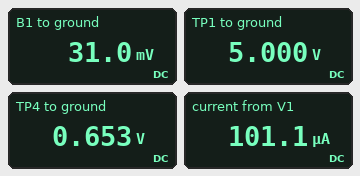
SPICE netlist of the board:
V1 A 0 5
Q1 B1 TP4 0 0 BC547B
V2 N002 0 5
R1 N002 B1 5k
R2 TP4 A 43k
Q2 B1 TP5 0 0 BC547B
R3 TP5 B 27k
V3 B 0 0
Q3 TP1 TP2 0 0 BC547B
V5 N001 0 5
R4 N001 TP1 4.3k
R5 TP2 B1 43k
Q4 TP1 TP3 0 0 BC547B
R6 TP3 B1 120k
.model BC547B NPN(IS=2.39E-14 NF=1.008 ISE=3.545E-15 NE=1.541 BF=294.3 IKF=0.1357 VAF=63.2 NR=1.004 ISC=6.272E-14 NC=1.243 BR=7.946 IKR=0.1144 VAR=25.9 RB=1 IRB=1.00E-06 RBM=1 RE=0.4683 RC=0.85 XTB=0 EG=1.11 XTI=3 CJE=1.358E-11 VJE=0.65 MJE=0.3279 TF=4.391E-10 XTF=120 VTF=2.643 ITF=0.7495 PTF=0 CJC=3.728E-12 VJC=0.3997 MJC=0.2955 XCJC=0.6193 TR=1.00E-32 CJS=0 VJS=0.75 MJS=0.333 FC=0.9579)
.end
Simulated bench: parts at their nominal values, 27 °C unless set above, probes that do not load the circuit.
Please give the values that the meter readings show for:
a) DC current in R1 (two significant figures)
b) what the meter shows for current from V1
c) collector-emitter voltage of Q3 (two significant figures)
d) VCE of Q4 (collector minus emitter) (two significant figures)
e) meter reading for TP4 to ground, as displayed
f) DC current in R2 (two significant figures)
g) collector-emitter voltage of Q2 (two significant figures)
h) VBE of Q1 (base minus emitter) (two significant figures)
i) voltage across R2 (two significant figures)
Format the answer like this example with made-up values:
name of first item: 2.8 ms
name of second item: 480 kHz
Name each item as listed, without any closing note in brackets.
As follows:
DC current in R1: 990 µA
what the meter shows for current from V1: 101.1 µA
collector-emitter voltage of Q3: 5.0 V
VCE of Q4 (collector minus emitter): 5.0 V
meter reading for TP4 to ground, as displayed: 0.653 V
DC current in R2: 100 µA
collector-emitter voltage of Q2: 31 mV
VBE of Q1 (base minus emitter): 650 mV
voltage across R2: 4.3 V
